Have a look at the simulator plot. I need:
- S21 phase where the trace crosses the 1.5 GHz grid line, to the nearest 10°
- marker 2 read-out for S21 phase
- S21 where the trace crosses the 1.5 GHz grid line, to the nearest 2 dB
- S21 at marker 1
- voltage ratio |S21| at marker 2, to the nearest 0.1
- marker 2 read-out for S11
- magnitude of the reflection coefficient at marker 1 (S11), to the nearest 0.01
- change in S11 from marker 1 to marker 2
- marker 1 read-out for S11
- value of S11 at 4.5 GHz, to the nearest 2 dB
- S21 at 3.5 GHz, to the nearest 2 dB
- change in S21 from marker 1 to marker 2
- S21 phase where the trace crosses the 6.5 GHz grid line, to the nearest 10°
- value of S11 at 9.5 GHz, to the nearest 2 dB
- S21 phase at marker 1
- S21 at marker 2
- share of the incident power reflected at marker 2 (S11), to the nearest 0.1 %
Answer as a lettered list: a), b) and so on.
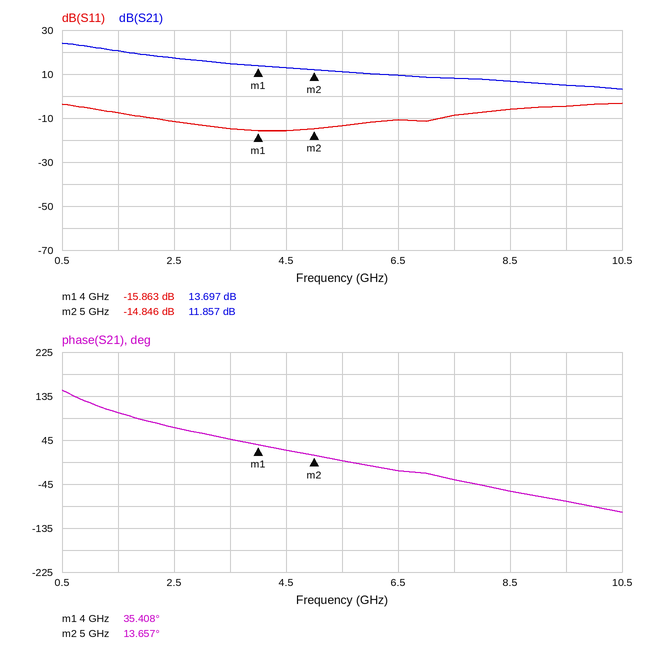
a) 100°
b) 13.657°
c) 20 dB
d) 13.697 dB
e) 3.9
f) -14.846 dB
g) 0.16
h) 1.017 dB
i) -15.863 dB
j) -16 dB
k) 14 dB
l) -1.840 dB
m) -20°
n) -4 dB
o) 35.408°
p) 11.857 dB
q) 3.3 %
